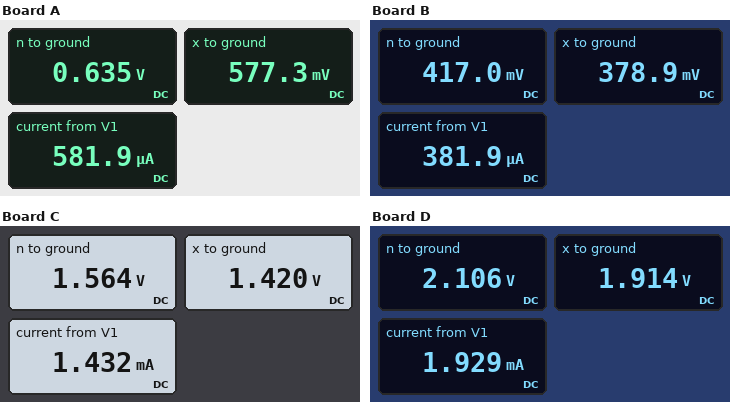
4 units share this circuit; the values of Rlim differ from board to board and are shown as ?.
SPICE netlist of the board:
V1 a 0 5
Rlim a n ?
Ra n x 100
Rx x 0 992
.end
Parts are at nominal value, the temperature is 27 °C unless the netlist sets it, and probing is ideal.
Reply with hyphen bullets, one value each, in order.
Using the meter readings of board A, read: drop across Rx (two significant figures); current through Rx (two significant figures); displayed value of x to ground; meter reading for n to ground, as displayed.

- 580 mV
- 580 µA
- 577.3 mV
- 0.635 V
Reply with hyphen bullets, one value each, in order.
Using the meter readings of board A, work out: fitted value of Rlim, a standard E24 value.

- 7.5 kΩ
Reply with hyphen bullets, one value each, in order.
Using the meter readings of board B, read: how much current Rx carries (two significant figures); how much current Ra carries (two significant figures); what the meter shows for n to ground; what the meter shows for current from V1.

- 380 µA
- 380 µA
- 417.0 mV
- 381.9 µA
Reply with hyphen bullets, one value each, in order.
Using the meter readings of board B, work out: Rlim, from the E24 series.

- 12 kΩ
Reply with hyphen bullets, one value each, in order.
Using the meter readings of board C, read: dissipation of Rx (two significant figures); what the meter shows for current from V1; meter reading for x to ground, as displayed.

- 2.0 mW
- 1.432 mA
- 1.420 V
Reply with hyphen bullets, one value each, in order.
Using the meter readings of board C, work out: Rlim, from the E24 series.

- 2.4 kΩ
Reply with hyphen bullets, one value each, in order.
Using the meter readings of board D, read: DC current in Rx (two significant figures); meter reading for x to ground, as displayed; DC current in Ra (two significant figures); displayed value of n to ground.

- 1.9 mA
- 1.914 V
- 1.9 mA
- 2.106 V
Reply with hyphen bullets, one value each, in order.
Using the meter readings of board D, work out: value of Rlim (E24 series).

- 1.5 kΩ
